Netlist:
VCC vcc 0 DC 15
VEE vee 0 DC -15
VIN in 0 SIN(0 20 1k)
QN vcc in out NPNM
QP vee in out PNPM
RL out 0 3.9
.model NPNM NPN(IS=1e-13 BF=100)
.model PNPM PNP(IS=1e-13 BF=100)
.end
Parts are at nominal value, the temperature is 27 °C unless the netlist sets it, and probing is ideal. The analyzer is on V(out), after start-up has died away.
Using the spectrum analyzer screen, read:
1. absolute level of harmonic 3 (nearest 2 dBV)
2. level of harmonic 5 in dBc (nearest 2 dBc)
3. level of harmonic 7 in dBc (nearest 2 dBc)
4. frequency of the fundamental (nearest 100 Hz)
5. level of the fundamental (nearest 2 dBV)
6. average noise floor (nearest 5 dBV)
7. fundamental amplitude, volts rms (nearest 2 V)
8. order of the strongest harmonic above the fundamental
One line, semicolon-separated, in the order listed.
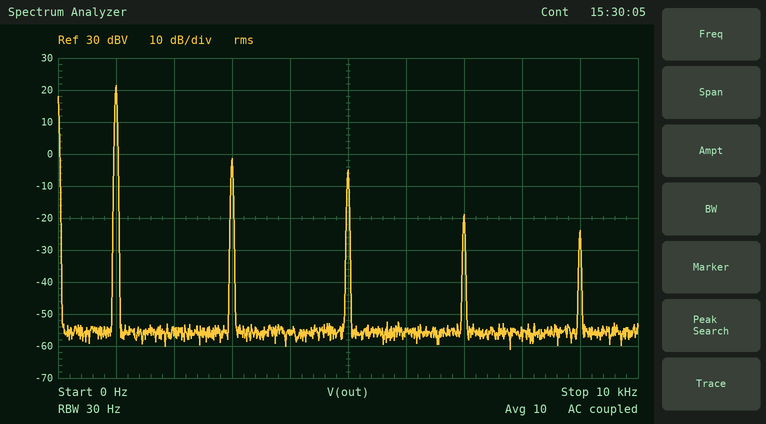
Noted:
-2 dBV; -26 dBc; -40 dBc; 1.0 kHz; 22 dBV; -55 dBV; 12 V; 3
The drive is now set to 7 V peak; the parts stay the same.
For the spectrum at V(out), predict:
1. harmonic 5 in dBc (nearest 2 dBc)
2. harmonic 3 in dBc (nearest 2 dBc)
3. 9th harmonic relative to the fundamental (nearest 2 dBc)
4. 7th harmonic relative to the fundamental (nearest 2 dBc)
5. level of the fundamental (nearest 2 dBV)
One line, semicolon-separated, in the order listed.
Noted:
-30 dBc; -26 dBc; -38 dBc; -34 dBc; 12 dBV
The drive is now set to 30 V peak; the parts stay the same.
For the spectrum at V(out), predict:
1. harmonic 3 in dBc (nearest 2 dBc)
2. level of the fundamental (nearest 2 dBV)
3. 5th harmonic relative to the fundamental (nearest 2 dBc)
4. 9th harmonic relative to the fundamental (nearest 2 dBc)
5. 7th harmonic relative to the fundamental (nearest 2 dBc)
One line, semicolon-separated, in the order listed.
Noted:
-14 dBc; 22 dBV; -32 dBc; -32 dBc; -30 dBc
